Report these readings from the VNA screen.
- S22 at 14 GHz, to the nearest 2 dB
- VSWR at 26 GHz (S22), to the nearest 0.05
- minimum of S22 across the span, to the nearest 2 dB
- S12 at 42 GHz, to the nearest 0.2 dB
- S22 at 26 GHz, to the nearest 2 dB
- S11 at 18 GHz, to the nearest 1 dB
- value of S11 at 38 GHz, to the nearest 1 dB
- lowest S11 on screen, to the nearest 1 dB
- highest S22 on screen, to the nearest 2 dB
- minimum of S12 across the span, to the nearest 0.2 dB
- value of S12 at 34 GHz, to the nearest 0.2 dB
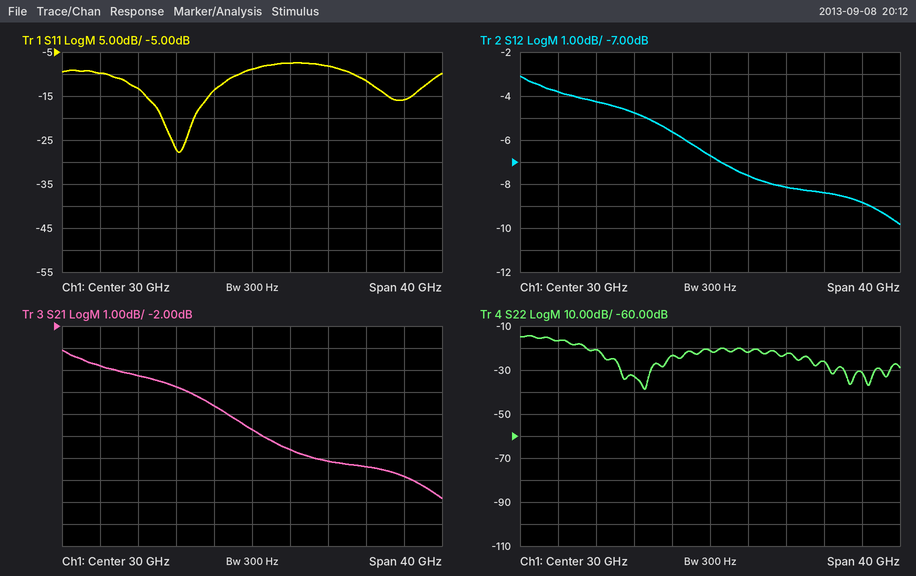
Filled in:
-16 dB
1.15
-38 dB
-8.4 dB
-24 dB
-13 dB
-8 dB
-28 dB
-14 dB
-9.8 dB
-7.6 dB
